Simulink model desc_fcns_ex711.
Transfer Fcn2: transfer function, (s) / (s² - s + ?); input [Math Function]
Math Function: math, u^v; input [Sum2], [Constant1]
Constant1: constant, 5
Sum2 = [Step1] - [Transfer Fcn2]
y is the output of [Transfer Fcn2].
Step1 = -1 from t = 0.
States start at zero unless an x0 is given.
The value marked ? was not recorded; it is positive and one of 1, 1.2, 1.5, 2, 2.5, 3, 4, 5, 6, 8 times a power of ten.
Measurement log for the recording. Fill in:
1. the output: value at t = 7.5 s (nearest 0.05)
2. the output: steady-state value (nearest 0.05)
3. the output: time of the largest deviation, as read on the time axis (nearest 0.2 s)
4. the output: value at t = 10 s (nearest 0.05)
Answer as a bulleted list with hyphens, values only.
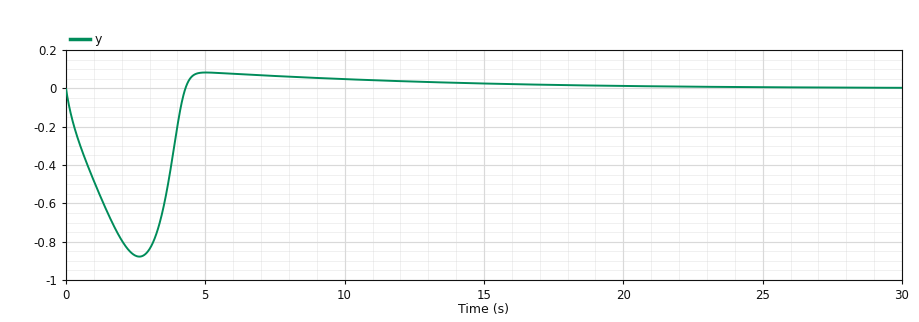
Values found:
- 0.05
- 0.00
- 2.6 s
- 0.05
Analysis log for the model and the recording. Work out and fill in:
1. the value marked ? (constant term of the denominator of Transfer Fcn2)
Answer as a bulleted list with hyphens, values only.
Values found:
- 0.6
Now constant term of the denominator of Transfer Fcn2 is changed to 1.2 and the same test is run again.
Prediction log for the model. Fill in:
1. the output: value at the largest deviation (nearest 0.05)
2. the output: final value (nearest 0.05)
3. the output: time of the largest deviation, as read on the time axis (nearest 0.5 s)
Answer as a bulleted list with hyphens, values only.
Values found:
- -0.45
- 0.00
- 1.5 s
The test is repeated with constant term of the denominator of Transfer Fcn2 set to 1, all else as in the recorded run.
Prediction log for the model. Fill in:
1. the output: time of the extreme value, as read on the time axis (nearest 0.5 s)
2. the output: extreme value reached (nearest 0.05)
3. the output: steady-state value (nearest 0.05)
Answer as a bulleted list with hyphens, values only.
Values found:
- 1.5 s
- -0.50
- 0.00
